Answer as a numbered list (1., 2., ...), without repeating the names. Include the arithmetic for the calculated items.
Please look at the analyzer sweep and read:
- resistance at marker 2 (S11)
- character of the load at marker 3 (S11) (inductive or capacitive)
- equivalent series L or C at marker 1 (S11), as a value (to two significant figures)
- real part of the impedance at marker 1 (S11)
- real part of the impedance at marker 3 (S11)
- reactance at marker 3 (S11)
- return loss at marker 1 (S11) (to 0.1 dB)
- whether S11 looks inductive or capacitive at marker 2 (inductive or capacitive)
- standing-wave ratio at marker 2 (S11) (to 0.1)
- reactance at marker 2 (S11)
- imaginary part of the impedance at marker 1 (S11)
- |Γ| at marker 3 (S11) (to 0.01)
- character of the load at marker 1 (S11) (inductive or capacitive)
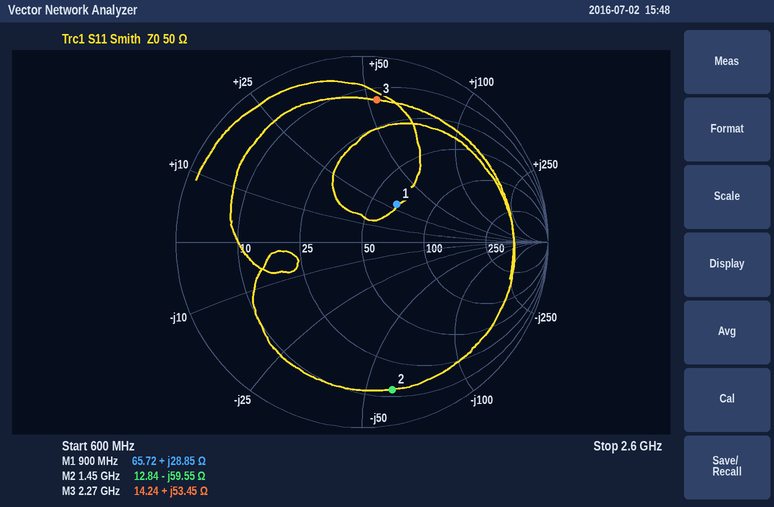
1. 12.84 Ω
2. inductive
3. L = 28.85 Ω/(2π × 900 MHz) ≈ 5.1 nH
4. 65.72 Ω
5. 14.24 Ω
6. +53.45 Ω
7. 11.2 dB
8. capacitive
9. 9.6
10. -59.55 Ω
11. +28.85 Ω
12. 0.77
13. inductive
